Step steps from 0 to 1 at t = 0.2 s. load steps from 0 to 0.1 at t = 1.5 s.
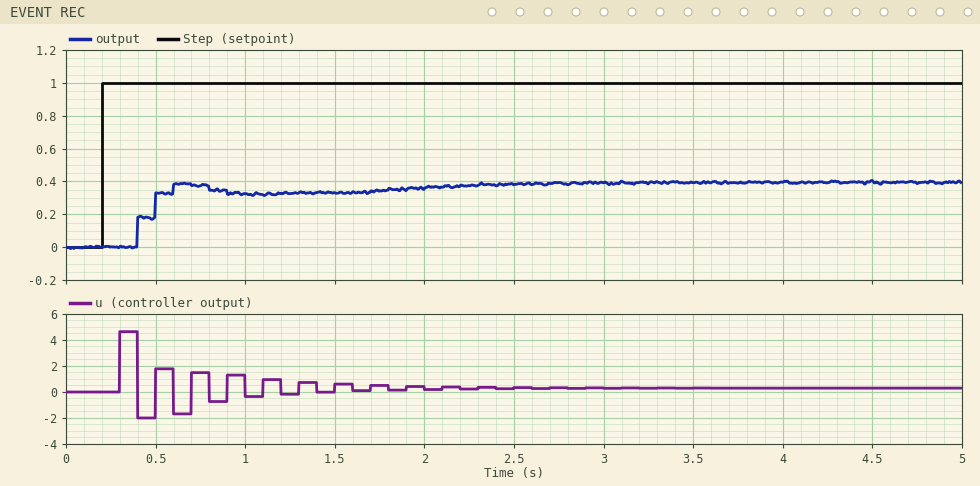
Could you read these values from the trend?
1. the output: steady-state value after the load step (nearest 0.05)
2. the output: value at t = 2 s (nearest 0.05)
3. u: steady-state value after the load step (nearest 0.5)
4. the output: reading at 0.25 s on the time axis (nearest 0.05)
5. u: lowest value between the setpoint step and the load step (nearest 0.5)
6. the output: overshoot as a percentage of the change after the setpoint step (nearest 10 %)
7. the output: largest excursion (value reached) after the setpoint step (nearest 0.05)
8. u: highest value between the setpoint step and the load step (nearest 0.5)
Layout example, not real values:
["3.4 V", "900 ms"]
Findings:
["0.40", "0.35", "0.5", "0.00", "-2.0", "20 %", "0.40", "4.5"]
